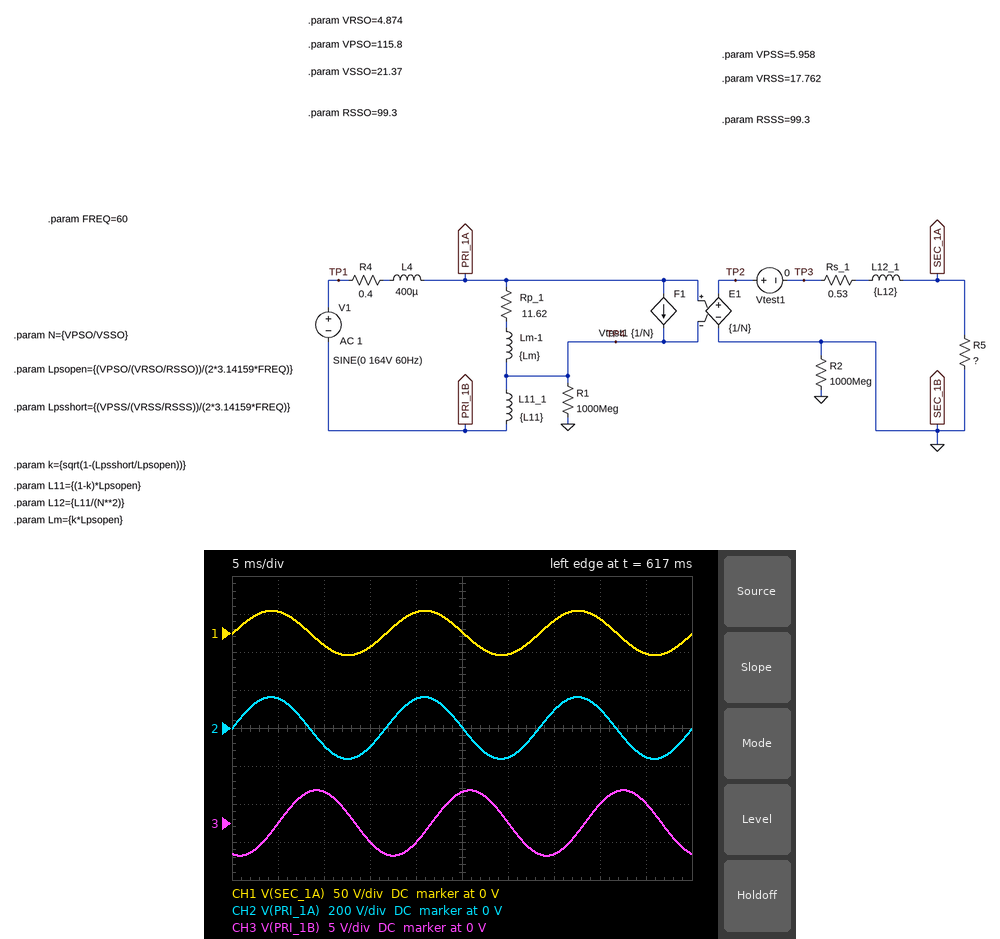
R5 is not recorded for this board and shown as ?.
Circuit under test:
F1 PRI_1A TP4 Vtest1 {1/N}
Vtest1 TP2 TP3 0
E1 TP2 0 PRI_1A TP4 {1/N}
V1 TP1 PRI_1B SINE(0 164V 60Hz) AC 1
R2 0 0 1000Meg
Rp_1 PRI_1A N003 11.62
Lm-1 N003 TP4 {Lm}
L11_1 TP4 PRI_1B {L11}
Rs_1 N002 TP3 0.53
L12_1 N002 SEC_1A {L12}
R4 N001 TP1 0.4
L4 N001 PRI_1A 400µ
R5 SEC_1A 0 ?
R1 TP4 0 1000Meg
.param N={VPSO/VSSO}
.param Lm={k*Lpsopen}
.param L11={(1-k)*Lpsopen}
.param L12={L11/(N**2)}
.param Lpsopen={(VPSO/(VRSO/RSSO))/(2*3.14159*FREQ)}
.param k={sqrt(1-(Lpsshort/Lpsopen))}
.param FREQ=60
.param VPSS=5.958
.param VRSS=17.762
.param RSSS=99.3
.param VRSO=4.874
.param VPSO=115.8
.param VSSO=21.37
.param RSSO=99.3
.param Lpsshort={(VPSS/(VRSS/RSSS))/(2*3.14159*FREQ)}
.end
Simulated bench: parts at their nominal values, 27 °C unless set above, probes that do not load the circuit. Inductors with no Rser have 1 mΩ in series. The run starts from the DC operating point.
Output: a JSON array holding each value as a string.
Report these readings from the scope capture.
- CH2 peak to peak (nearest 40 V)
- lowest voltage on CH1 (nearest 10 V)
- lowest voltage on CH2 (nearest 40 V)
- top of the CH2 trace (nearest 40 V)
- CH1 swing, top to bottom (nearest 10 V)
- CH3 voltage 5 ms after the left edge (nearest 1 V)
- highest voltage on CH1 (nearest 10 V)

["320 V", "-30 V", "-160 V", "160 V", "60 V", "0 V", "30 V"]
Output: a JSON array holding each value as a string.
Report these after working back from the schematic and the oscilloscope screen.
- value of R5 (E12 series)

["22 Ω"]
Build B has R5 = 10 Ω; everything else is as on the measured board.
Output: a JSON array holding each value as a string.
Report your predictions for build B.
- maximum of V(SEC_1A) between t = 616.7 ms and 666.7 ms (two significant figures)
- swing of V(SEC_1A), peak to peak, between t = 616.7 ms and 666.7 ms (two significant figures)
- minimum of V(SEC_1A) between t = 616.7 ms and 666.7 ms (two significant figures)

["28 V", "57 V", "-28 V"]
